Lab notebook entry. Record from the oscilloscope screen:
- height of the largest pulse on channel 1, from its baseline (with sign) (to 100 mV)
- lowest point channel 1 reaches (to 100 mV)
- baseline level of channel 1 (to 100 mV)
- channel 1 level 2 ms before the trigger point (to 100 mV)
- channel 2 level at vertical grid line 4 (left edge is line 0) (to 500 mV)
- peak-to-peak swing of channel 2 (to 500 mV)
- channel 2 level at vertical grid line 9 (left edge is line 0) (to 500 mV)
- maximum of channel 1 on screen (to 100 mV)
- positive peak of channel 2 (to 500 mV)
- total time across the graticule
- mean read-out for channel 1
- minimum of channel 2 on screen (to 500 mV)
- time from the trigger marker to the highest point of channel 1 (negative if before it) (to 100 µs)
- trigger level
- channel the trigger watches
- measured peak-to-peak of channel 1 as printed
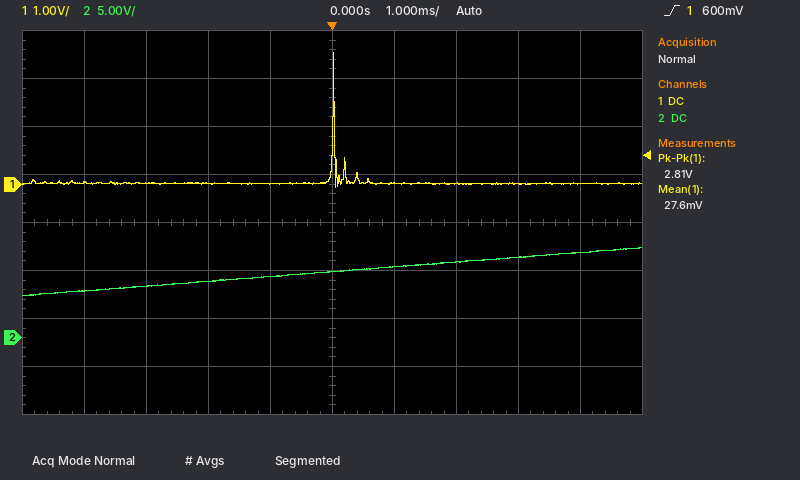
+2.7 V
-100 mV
0.0 V
0.0 V
6.5 V
5.0 V
9.0 V
2.7 V
9.5 V
10 ms
27.6 mV
4.5 V
0.0 ms
600 mV
channel 1
2.81 V
